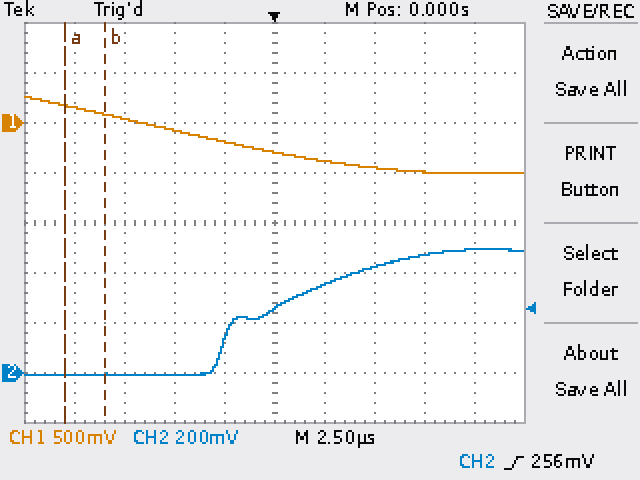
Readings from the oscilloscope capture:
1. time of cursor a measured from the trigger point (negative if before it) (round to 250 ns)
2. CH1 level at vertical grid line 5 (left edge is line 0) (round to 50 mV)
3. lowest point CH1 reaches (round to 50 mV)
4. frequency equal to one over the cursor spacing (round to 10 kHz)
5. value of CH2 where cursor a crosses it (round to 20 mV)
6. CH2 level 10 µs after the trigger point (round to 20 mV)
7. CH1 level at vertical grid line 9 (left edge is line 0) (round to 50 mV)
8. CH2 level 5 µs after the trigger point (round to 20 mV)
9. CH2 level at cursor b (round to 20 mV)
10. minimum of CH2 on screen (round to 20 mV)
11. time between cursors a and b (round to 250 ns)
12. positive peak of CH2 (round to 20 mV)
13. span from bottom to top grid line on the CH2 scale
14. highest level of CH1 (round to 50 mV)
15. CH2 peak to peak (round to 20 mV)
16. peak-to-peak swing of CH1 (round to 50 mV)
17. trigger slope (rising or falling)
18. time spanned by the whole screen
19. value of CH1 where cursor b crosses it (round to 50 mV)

-10.50 µs
-300 mV
-500 mV
500 kHz
0 mV
500 mV
-500 mV
420 mV
0 mV
0 mV
2.00 µs
500 mV
1.6 V
250 mV
500 mV
750 mV
rising
25 µs
100 mV
